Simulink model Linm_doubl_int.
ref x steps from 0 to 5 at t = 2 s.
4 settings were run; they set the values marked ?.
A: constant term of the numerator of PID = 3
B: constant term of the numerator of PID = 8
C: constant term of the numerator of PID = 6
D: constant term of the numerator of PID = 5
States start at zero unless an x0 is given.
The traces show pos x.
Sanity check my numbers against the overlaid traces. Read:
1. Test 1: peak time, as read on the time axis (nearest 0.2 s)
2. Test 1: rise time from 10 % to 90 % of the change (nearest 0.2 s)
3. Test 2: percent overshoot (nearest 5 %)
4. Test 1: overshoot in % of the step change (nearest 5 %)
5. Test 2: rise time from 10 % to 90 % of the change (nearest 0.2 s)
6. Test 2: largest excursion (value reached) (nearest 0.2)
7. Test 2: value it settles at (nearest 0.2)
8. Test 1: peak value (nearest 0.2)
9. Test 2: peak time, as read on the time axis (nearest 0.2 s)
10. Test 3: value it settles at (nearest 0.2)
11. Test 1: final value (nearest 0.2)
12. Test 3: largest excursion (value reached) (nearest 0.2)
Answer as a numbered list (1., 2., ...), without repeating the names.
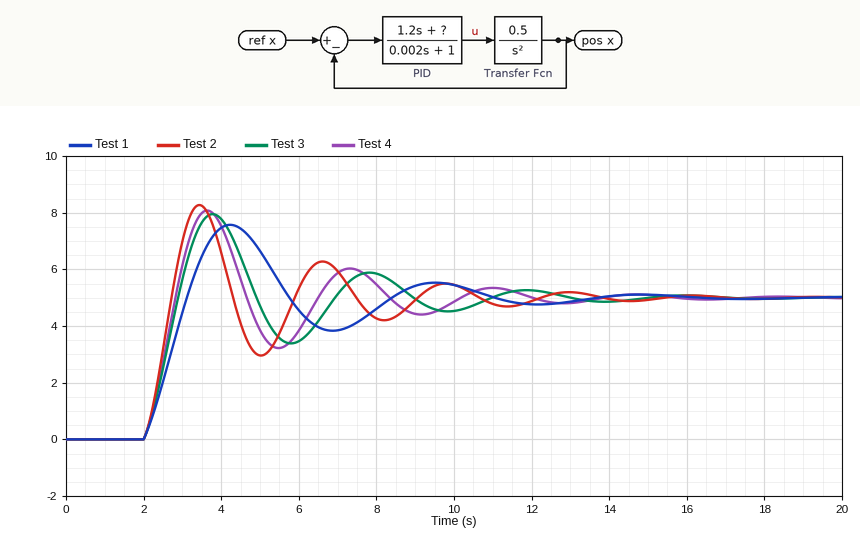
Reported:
1. 4.2 s
2. 0.8 s
3. 65 %
4. 50 %
5. 0.6 s
6. 8.2
7. 5.0
8. 7.6
9. 3.4 s
10. 5.0
11. 5.0
12. 8.0
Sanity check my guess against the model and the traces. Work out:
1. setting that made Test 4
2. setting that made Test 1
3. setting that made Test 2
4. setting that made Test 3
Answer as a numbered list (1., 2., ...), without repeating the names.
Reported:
1. C
2. A
3. B
4. D
